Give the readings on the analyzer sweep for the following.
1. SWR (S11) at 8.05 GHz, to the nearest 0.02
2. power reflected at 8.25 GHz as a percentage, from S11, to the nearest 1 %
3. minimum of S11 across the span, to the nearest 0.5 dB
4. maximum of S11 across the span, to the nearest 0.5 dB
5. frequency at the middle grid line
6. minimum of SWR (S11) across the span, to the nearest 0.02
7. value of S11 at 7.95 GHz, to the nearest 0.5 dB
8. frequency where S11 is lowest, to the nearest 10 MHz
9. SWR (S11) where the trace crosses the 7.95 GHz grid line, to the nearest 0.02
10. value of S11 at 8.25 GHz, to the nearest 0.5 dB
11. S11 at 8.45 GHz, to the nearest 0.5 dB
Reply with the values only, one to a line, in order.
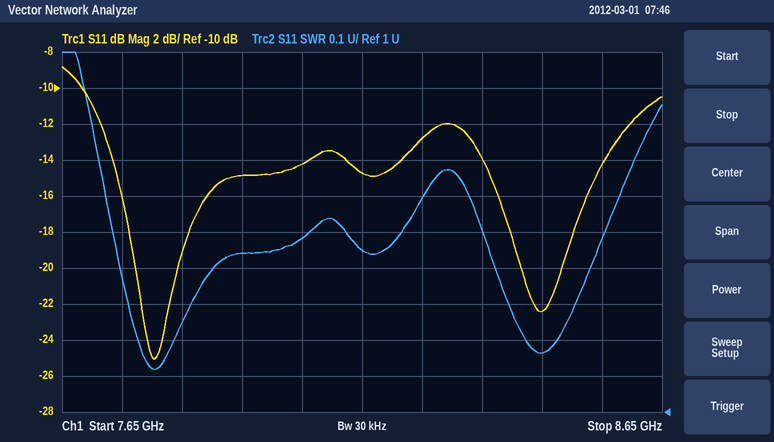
1.48
5 %
-25.0 dB
-9.0 dB
8.15 GHz
1.12
-15.0 dB
7.80 GHz
1.44
-13.0 dB
-22.5 dB
